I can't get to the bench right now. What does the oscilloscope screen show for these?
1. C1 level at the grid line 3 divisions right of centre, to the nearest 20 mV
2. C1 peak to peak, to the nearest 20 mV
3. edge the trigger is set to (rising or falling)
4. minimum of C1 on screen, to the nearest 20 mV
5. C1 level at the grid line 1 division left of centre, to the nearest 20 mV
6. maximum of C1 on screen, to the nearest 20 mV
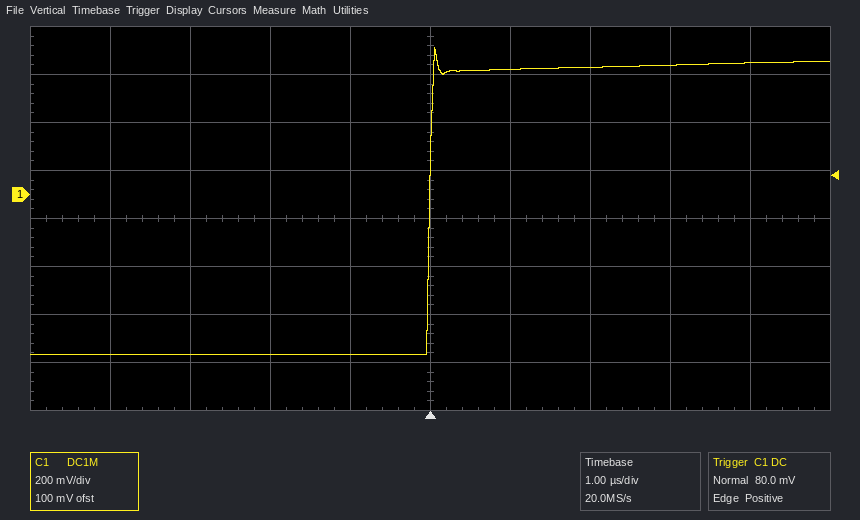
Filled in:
540 mV
1.28 V
rising
-660 mV
-660 mV
620 mV
